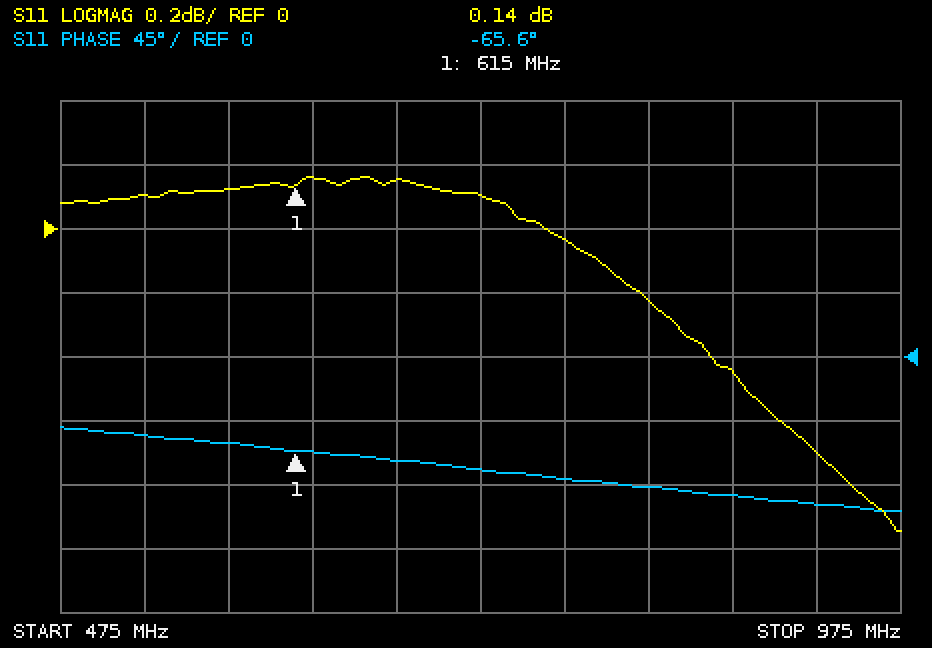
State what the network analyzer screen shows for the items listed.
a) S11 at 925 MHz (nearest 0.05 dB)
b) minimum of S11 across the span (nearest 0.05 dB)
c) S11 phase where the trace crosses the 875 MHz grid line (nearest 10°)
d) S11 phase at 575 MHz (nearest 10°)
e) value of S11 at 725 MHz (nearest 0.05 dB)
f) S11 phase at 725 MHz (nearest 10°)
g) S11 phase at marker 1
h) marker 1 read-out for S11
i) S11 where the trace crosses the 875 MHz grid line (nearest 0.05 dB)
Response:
-0.70 dB
-0.95 dB
-100°
-60°
0.10 dB
-80°
-65.6°
0.14 dB
-0.45 dB
